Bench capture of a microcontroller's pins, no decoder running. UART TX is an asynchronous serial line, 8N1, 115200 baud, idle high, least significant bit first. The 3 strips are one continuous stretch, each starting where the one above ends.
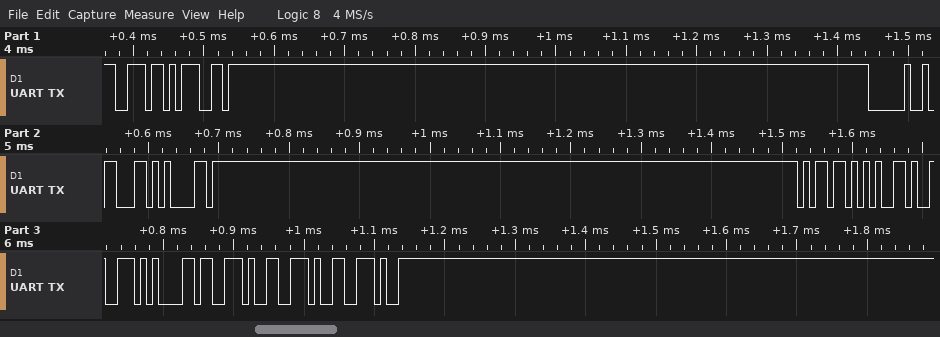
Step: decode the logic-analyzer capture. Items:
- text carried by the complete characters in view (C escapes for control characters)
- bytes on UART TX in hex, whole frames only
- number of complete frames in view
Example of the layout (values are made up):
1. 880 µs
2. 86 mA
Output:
1. "ng camera..."
2. 0x6E 0x67 0x20 0x63 0x61 0x6D 0x65 0x72 0x61 0x2E 0x2E 0x2E
3. 12
